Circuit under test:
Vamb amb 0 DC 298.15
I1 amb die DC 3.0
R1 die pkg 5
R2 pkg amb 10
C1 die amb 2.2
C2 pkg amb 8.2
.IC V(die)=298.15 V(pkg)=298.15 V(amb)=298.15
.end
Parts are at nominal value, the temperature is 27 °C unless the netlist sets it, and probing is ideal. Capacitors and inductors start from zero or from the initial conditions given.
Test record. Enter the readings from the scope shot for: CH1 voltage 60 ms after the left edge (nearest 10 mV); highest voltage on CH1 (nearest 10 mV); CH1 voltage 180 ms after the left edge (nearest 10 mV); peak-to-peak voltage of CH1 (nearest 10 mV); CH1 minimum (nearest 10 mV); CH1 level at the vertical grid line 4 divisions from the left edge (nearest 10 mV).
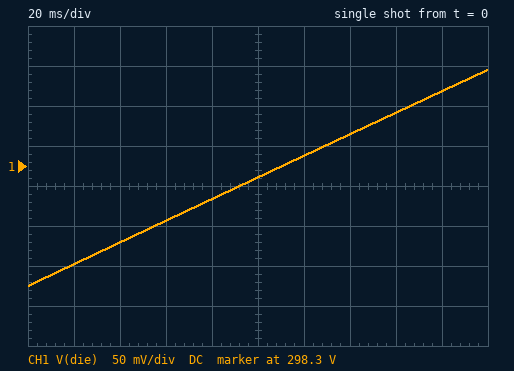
298.23 V
298.42 V
298.39 V
270 mV
298.15 V
298.26 V
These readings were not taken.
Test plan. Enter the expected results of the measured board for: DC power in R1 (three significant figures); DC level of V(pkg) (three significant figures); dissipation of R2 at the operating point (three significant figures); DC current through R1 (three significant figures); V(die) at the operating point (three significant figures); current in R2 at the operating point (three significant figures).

45.0 W
328 V
90.0 W
3.00 A
343 V
3.00 A
